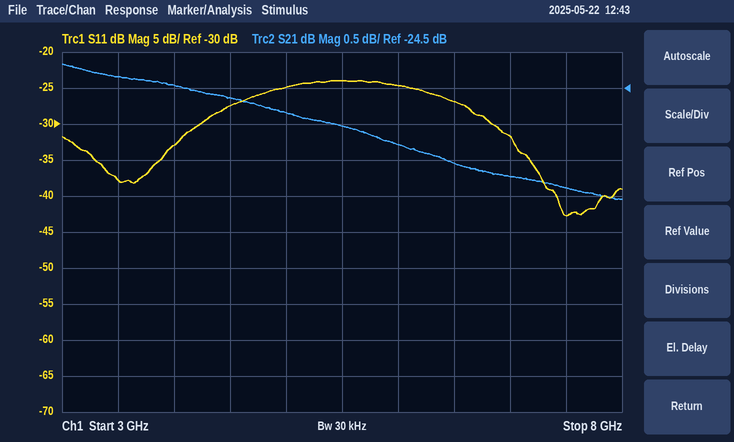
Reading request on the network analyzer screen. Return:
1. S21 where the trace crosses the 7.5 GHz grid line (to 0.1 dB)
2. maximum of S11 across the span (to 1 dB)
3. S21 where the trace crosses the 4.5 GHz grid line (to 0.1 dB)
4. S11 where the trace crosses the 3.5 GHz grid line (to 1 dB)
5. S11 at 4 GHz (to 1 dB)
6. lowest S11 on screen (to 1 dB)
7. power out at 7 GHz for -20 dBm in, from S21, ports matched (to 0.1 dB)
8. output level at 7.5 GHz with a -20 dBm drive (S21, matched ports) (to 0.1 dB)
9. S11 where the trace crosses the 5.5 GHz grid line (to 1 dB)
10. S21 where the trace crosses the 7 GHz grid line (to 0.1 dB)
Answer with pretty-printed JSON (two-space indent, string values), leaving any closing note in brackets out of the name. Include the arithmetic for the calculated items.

{
  "S21 where the trace crosses the 7.5 GHz grid line": "-25.9 dB",
  "maximum of S11 across the span": "-24 dB",
  "S21 where the trace crosses the 4.5 GHz grid line": "-24.6 dB",
  "S11 where the trace crosses the 3.5 GHz grid line": "-38 dB",
  "S11 at 4 GHz": "-33 dB",
  "lowest S11 on screen": "-43 dB",
  "power out at 7 GHz for -20 dBm in, from S21, ports matched": "-20 dBm + (-25.7 dB) = -45.7 dBm",
  "output level at 7.5 GHz with a -20 dBm drive (S21, matched ports)": "-20 dBm + (-25.9 dB) = -45.9 dBm",
  "S11 where the trace crosses the 5.5 GHz grid line": "-24 dB",
  "S21 where the trace crosses the 7 GHz grid line": "-25.7 dB"
}
